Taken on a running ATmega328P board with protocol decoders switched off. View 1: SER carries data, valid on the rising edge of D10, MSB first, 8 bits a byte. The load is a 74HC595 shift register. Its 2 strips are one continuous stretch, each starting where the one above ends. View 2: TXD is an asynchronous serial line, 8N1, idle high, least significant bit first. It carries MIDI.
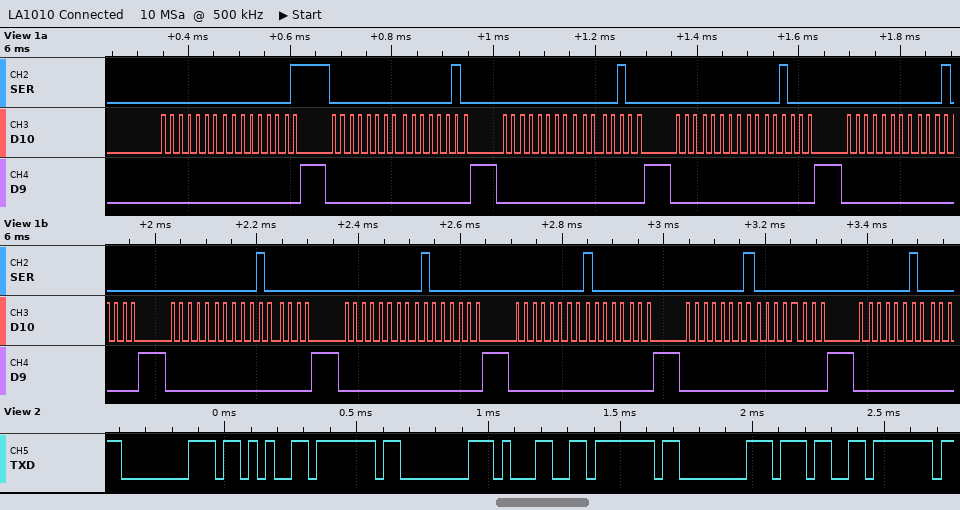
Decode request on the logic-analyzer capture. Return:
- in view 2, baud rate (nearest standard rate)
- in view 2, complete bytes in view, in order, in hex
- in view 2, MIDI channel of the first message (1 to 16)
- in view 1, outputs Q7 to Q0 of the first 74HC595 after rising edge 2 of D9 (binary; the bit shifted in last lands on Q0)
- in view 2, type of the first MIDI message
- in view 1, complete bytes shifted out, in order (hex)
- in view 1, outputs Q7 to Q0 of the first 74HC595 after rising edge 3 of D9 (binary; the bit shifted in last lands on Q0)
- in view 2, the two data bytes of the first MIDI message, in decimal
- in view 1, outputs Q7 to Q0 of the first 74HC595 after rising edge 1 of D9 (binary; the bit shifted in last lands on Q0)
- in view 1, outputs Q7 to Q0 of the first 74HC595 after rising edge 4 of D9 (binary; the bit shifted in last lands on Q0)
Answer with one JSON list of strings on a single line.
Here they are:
["31250 baud", "80 2B 7F 80 31 7F 80 37 7F", "1", "00000010", "Note Off", "00 01 00 02 00 04 00 08 00 10 00 20 00 40 00 80 01 00 02", "00000100", "43, 127", "00000001", "00001000"]
